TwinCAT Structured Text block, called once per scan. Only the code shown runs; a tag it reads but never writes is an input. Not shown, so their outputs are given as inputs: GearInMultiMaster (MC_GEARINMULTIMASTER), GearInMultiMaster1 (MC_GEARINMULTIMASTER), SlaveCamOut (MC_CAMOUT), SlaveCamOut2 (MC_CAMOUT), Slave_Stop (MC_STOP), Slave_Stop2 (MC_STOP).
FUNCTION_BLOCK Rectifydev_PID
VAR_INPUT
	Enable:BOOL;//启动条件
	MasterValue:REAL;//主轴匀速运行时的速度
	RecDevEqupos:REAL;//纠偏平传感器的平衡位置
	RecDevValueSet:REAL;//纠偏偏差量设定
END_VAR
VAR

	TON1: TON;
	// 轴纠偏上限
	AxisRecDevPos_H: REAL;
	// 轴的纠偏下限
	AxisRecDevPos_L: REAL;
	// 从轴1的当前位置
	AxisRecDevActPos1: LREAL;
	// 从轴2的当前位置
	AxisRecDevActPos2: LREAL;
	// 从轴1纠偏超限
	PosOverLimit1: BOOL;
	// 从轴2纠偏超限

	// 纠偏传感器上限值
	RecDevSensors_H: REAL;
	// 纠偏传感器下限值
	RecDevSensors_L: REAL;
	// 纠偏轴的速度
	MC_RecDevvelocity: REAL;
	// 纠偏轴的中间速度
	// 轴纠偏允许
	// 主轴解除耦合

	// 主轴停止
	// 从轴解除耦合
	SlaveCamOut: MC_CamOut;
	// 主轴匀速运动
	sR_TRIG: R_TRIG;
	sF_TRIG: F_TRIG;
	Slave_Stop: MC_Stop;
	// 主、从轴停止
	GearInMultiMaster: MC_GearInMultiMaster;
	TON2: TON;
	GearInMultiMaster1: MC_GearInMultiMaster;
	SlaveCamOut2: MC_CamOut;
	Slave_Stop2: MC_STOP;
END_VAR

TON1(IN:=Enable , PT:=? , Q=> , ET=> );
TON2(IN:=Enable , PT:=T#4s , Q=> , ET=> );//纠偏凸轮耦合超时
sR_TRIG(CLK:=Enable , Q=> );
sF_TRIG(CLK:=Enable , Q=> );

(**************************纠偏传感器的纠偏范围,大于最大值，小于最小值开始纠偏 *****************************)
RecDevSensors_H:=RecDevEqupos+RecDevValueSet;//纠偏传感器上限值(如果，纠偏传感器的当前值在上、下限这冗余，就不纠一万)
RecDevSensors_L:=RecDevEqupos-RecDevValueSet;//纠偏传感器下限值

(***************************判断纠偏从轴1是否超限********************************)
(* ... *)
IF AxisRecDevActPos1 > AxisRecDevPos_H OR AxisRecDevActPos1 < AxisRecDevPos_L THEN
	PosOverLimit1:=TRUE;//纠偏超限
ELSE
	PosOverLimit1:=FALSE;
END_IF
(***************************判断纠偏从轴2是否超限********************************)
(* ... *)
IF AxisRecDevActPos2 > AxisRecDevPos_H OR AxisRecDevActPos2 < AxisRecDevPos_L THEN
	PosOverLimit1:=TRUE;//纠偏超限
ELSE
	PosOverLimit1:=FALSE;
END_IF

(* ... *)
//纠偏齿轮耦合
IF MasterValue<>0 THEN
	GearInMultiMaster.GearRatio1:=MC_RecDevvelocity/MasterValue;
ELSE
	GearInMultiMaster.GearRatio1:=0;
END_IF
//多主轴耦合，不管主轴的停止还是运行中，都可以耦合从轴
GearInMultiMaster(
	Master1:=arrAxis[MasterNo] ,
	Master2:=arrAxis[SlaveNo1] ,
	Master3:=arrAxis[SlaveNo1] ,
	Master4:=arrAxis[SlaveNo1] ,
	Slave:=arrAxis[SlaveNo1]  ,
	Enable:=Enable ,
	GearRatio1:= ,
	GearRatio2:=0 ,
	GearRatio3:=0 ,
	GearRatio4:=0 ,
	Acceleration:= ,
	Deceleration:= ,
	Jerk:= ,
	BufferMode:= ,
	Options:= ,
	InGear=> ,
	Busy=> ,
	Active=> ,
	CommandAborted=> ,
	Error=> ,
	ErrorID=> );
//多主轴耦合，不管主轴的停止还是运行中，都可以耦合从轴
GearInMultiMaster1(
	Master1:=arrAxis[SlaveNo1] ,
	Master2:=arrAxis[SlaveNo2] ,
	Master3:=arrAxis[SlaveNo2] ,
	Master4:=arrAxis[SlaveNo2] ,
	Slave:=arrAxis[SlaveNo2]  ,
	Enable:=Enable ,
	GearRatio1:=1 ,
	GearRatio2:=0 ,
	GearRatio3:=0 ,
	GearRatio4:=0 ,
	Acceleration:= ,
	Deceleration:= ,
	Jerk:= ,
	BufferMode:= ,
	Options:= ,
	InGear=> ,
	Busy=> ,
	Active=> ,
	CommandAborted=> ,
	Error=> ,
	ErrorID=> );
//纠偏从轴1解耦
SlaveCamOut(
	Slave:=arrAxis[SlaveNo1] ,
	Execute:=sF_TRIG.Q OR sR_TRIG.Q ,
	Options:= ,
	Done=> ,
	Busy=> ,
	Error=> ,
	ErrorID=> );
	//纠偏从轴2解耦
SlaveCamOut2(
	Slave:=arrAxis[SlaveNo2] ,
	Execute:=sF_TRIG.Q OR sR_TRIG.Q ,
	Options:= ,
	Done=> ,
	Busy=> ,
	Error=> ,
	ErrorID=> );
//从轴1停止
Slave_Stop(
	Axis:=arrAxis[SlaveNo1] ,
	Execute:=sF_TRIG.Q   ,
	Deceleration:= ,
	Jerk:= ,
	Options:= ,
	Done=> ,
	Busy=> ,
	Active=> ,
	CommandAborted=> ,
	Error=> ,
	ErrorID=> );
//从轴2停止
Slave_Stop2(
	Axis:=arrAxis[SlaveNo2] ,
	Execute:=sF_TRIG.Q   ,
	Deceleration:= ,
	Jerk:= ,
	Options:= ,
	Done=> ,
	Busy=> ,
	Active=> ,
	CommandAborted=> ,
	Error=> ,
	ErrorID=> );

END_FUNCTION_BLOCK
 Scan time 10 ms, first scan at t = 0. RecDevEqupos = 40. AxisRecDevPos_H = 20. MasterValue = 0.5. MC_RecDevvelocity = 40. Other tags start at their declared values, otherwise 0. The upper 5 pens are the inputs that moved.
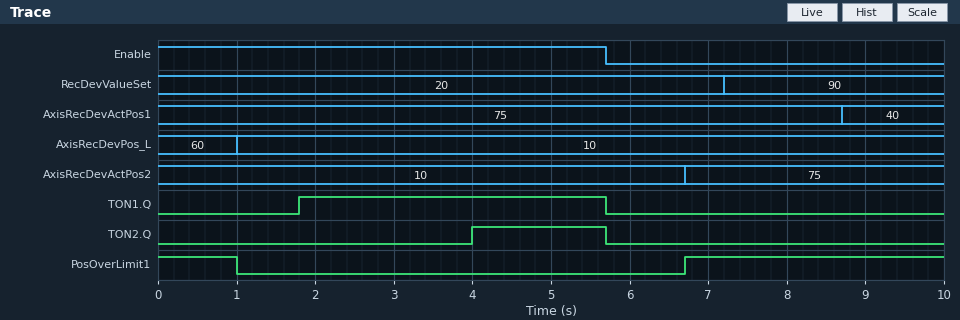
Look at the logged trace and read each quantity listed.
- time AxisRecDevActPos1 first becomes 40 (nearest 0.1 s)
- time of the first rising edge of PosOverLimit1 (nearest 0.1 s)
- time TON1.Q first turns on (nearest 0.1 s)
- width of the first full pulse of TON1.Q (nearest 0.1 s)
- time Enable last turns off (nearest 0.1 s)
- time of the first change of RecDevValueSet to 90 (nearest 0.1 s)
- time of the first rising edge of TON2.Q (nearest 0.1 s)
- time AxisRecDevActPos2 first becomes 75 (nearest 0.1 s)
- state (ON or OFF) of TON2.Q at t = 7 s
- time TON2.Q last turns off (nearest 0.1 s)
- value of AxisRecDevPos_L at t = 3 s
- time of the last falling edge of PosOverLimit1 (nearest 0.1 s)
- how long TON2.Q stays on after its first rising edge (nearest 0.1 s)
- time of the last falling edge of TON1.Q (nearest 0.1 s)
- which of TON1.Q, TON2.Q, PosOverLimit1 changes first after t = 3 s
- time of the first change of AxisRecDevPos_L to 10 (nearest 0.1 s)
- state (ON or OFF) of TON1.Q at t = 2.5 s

8.7 s
6.7 s
1.8 s
3.9 s
5.7 s
7.2 s
4.0 s
6.7 s
OFF
5.7 s
10
1.0 s
1.7 s
5.7 s
TON2.Q
1.0 s
ON
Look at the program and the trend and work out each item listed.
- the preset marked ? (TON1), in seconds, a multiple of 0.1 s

1.8 s
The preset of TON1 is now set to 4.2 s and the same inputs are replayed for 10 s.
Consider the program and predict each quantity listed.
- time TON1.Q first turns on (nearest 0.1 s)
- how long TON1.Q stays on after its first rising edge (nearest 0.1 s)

4.2 s
1.5 s
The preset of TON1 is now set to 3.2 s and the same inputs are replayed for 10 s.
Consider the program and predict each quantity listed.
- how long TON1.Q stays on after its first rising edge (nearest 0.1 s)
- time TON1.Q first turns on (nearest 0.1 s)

2.5 s
3.2 s
